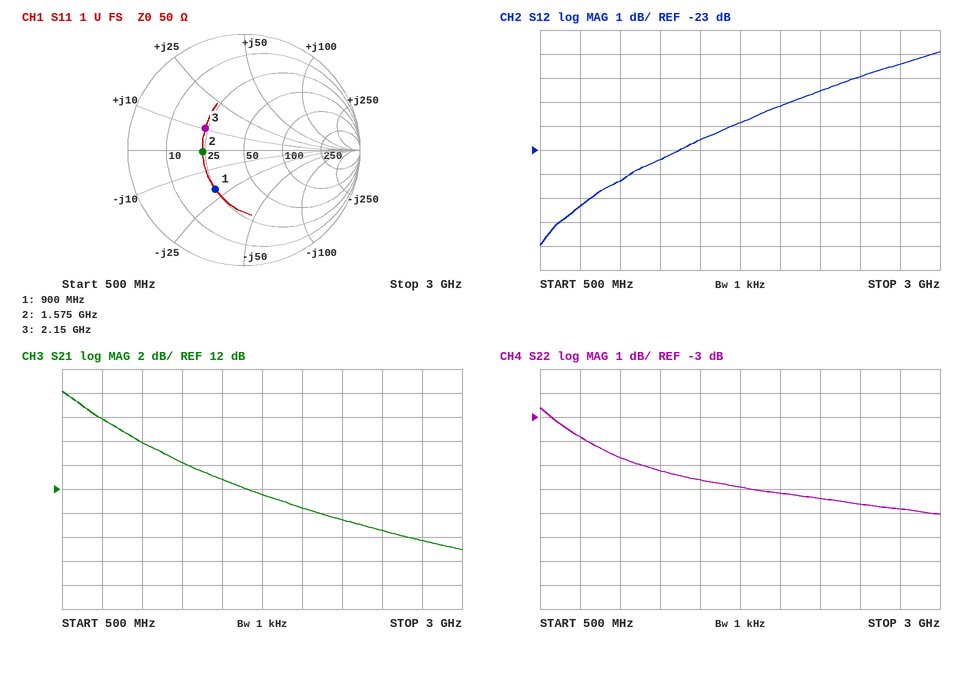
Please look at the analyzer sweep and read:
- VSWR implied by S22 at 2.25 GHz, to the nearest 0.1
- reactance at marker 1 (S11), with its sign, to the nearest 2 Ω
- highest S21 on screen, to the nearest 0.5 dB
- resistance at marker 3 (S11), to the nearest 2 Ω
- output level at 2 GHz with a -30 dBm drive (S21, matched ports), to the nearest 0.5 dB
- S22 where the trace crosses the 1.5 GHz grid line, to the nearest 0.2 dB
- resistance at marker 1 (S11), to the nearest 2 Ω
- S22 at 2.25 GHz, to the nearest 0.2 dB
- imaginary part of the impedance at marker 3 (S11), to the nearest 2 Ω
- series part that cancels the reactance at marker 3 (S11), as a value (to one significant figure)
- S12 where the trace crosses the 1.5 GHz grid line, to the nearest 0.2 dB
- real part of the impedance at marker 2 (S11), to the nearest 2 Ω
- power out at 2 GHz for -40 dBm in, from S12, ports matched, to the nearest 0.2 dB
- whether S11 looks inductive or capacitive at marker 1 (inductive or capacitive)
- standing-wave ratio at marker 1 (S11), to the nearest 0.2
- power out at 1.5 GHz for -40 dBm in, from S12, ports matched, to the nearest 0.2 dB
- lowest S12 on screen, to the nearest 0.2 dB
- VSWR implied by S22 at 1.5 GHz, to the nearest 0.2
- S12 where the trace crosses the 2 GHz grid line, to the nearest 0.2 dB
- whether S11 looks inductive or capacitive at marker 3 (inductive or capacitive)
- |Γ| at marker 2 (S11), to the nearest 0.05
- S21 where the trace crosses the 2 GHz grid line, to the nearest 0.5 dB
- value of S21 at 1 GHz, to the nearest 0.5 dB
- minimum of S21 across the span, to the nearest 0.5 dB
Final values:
2.8
-20 Ω
20.0 dB
24 Ω
-19.5 dBm
-5.6 dB
24 Ω
-6.4 dB
+10 Ω
7 pF
-22.6 dB
24 Ω
-61.2 dBm
capacitive
2.4
-62.6 dBm
-27.0 dB
3.2
-21.2 dB
inductive
0.35
10.5 dB
16.0 dB
7.0 dB
